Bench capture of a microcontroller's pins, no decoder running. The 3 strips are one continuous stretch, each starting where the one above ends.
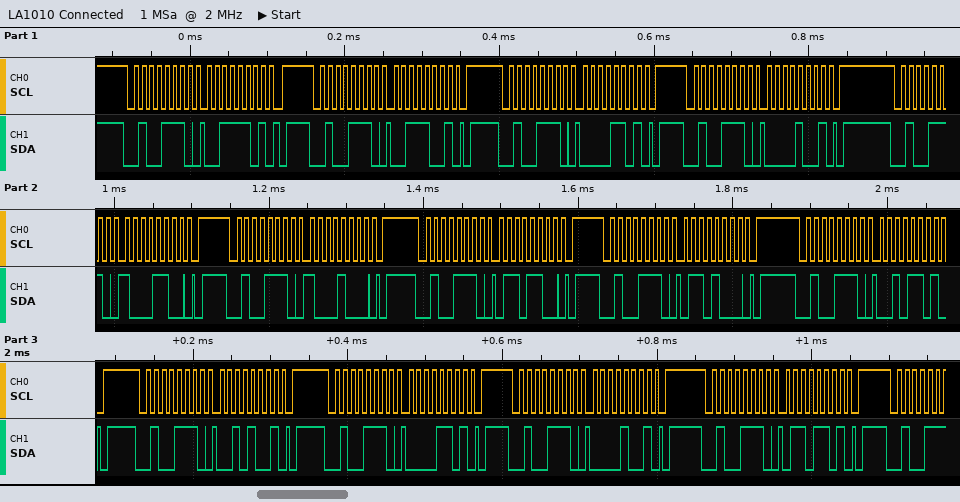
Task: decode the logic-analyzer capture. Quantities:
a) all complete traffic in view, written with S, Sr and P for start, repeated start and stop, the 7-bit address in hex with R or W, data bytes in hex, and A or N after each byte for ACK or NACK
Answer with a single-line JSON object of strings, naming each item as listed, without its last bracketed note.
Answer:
{"all complete traffic in view, written with S, Sr and P for start, repeated start and stop, the 7-bit address in hex with R or W, data bytes in hex, and A or N after each byte for ACK or NACK": "S 27W A 3D A P S 27W A 39 A P S 27W A 0D A P S 27W A 09 A P S 27W A 8C A P S 27W A 88 A P S 27W A 6C A P S 27W A 68 A P S 27W A 2D A P S 27W A 29 A P S 27W A 0D A P S 27W A 09 A P S 27W A 6D A P"}
